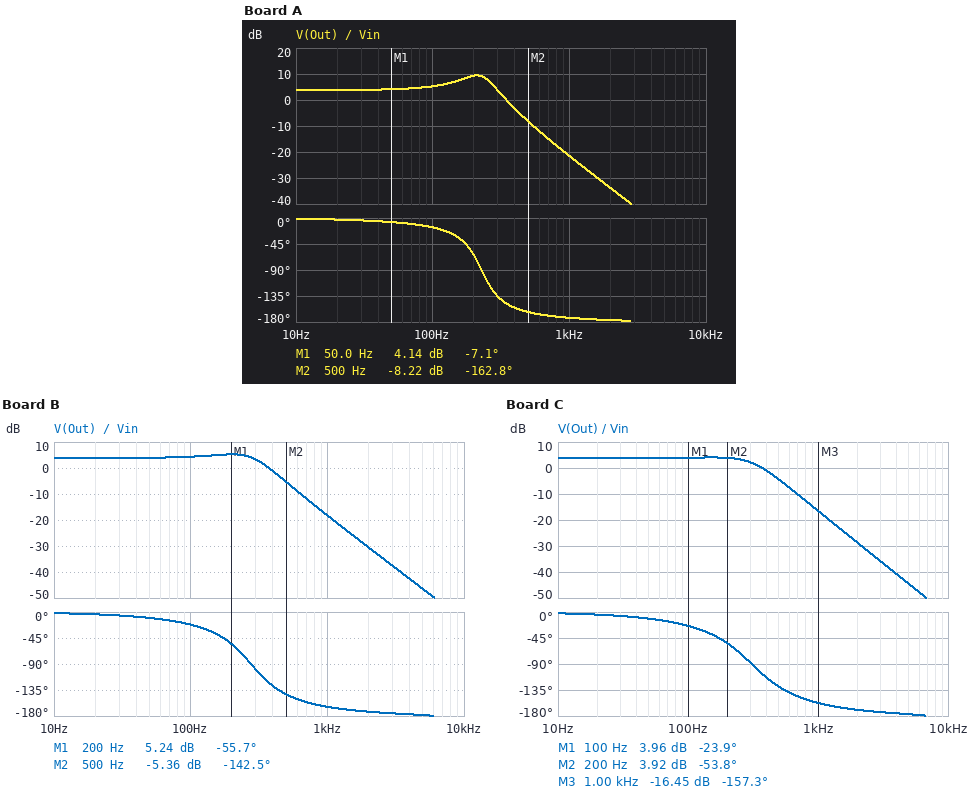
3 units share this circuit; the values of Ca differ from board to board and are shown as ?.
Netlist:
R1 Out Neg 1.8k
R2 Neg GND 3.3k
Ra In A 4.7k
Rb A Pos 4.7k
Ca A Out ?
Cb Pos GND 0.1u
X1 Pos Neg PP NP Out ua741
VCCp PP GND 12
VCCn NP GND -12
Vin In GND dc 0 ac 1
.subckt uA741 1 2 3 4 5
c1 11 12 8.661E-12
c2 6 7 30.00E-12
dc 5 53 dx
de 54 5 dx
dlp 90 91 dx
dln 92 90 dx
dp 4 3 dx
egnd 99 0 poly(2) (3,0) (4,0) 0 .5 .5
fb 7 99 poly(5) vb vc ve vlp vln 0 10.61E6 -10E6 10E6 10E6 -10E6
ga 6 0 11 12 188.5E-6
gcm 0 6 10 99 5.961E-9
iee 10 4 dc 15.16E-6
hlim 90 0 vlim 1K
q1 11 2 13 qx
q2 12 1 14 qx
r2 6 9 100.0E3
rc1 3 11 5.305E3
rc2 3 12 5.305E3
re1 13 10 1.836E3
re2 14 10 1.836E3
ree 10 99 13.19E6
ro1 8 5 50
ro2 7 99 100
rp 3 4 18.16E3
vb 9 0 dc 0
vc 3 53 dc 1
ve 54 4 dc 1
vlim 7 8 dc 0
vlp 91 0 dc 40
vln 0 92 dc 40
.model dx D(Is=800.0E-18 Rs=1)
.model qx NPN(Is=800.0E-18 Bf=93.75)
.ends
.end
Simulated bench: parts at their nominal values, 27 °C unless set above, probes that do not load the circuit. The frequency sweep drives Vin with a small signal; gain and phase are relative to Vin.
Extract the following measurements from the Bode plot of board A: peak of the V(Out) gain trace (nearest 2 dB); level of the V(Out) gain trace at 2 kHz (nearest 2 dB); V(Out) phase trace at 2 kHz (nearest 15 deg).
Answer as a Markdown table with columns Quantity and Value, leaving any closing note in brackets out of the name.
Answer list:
| Quantity | Value |
|---|---|
| peak of the V(Out) gain trace | 10 dB |
| level of the V(Out) gain trace at 2 kHz | -34 dB |
| V(Out) phase trace at 2 kHz | -180 deg |
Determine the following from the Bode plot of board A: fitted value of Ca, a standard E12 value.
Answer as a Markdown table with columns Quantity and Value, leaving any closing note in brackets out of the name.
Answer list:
| Quantity | Value |
|---|---|
| fitted value of Ca, a standard E12 value | 220 nF |
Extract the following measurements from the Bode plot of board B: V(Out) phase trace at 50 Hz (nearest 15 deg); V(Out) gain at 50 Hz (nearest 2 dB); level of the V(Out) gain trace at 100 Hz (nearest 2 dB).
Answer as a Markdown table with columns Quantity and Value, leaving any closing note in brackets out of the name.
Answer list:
| Quantity | Value |
|---|---|
| V(Out) phase trace at 50 Hz | -15 deg |
| V(Out) gain at 50 Hz | 4 dB |
| level of the V(Out) gain trace at 100 Hz | 4 dB |
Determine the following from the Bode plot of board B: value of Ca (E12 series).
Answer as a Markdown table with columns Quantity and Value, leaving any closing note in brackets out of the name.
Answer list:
| Quantity | Value |
|---|---|
| value of Ca | 150 nF |
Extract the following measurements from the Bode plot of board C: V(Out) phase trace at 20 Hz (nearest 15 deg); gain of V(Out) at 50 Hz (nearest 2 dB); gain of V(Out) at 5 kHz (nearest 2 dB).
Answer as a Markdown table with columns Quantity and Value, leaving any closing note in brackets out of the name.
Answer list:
| Quantity | Value |
|---|---|
| V(Out) phase trace at 20 Hz | 0 deg |
| gain of V(Out) at 50 Hz | 4 dB |
| gain of V(Out) at 5 kHz | -44 dB |
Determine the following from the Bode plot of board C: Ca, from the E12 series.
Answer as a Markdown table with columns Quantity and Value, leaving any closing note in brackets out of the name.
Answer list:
| Quantity | Value |
|---|---|
| Ca, from the E12 series | 120 nF |
